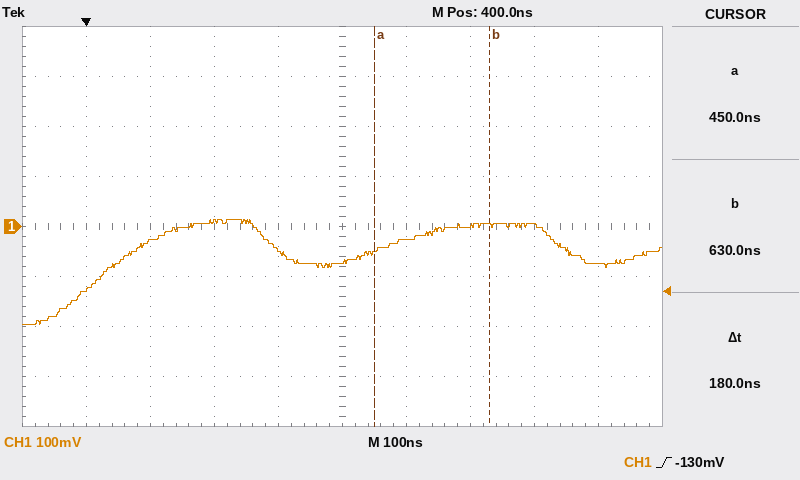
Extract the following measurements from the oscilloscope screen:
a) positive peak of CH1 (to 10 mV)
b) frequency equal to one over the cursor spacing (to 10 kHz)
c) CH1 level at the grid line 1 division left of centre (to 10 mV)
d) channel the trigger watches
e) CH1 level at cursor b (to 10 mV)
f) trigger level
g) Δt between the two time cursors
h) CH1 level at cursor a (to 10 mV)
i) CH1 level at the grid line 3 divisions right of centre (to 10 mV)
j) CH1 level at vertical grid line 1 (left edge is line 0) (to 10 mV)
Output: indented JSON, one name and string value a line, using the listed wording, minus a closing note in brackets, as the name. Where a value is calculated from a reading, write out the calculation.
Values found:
{
  "positive peak of CH1": "10 mV",
  "frequency equal to one over the cursor spacing": "1 / 180 ns ≈ 5.56 MHz",
  "CH1 level at the grid line 1 division left of centre": "-50 mV",
  "channel the trigger watches": "CH1",
  "CH1 level at cursor b": "0 mV",
  "trigger level": "-130 mV",
  "Δt between the two time cursors": "180 ns",
  "CH1 level at cursor a": "-50 mV",
  "CH1 level at the grid line 3 divisions right of centre": "0 mV",
  "CH1 level at vertical grid line 1 (left edge is line 0)": "-130 mV"
}
